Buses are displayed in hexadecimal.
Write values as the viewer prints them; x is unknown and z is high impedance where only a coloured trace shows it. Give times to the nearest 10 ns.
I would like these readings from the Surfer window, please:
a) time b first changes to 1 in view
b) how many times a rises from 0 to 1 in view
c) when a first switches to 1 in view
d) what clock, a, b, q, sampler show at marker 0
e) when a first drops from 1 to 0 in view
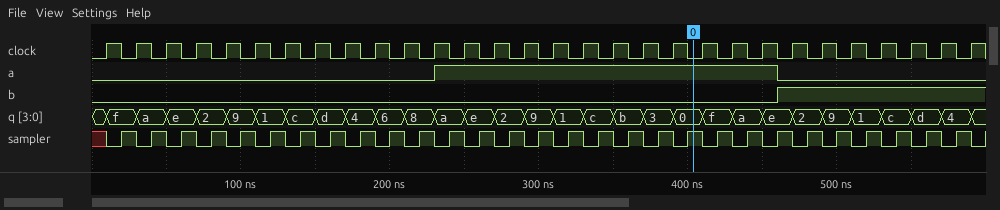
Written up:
460 ns
1
230 ns
clock=0, a=1, b=0, q=0, sampler=1
460 ns
